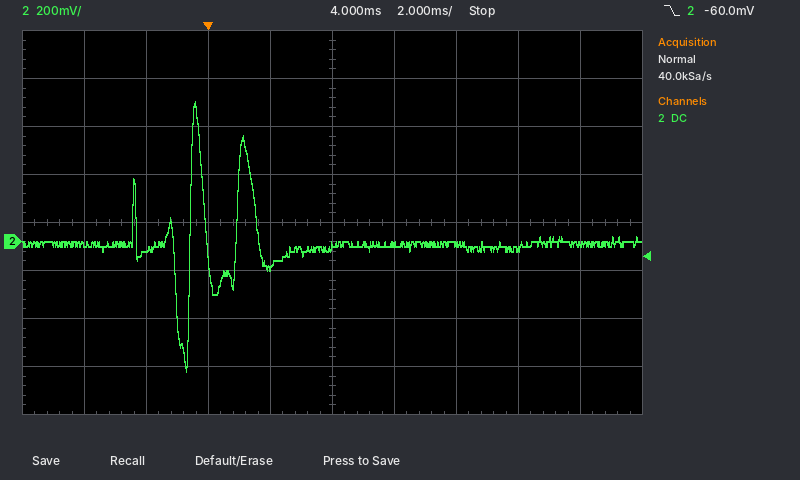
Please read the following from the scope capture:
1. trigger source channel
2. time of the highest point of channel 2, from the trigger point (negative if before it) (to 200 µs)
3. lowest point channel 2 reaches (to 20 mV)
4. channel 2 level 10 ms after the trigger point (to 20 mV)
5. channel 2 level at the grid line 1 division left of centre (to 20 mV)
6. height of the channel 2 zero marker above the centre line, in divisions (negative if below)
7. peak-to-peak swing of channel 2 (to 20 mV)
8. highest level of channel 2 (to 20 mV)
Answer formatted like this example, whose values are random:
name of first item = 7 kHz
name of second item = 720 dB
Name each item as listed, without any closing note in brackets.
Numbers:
trigger source channel = channel 2
time of the highest point of channel 2, from the trigger point (negative if before it) = -400 µs
lowest point channel 2 reaches = -540 mV
channel 2 level 10 ms after the trigger point = -20 mV
channel 2 level at the grid line 1 division left of centre = -100 mV
height of the channel 2 zero marker above the centre line, in divisions = -0.4 div
peak-to-peak swing of channel 2 = 1.12 V
highest level of channel 2 = 580 mV
